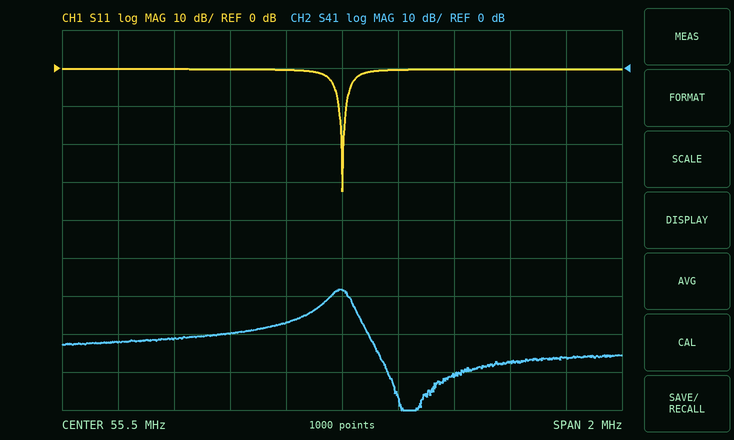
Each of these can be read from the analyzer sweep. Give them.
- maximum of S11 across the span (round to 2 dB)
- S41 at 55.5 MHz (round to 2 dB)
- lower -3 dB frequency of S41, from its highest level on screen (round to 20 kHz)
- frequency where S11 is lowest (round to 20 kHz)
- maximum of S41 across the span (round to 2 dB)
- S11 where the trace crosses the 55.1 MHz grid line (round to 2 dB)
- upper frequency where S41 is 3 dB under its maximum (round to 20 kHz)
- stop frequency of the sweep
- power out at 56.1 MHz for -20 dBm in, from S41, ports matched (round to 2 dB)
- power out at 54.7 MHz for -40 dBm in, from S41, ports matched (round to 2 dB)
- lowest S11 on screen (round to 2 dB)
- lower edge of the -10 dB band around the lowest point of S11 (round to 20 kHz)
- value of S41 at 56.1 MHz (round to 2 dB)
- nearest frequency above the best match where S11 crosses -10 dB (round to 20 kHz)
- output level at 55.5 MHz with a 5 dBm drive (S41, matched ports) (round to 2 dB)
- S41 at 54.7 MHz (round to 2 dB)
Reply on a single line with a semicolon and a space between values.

0 dB; -58 dB; 55.44 MHz; 55.50 MHz; -58 dB; 0 dB; 55.54 MHz; 56.5 MHz; -98 dBm; -112 dBm; -32 dB; 55.48 MHz; -78 dB; 55.52 MHz; -54 dBm; -72 dB
